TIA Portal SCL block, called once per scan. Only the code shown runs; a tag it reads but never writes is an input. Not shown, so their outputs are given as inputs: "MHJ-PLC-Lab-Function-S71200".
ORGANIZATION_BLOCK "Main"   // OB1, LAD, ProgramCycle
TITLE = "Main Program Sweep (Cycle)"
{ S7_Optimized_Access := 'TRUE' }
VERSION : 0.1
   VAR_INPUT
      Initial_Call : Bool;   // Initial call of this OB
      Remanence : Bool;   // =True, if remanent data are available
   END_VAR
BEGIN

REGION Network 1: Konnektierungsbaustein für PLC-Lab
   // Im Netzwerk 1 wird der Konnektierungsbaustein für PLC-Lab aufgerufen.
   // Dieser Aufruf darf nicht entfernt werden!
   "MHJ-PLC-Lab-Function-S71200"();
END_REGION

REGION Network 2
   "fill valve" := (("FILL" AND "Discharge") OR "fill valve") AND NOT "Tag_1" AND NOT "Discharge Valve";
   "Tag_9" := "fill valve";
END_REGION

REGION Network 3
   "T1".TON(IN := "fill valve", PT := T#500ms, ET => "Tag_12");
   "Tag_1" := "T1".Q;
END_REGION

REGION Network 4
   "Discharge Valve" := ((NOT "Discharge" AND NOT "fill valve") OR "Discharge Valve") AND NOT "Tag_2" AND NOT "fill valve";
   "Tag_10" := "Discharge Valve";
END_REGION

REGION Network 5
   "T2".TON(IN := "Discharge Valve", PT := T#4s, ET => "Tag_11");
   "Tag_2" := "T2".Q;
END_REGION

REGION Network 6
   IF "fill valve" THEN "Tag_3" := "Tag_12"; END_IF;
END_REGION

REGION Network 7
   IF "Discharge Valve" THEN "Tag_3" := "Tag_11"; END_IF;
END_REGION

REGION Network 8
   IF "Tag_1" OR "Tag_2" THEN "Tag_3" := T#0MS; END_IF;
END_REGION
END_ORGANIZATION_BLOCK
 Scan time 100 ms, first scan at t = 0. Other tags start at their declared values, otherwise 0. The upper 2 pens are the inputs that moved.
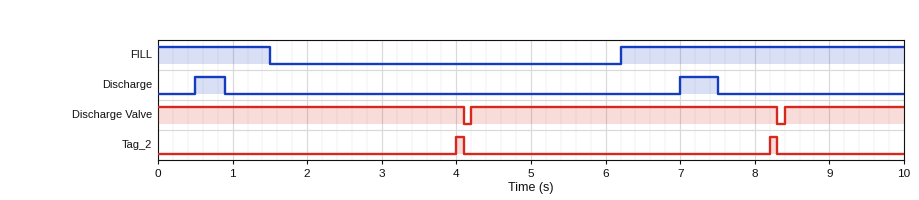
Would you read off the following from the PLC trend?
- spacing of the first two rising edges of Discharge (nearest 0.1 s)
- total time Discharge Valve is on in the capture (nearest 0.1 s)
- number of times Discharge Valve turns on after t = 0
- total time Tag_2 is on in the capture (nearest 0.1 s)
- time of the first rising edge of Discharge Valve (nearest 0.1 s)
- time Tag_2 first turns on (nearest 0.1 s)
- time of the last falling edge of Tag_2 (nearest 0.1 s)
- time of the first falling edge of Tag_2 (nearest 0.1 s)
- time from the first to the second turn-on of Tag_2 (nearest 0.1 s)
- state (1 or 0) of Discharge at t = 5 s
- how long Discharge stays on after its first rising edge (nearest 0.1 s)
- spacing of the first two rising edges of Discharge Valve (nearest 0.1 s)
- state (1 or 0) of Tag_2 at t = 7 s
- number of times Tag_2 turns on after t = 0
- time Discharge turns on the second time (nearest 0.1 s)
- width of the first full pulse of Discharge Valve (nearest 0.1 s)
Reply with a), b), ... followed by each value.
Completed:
a) 6.5 s
b) 9.8 s
c) 2
d) 0.2 s
e) 4.2 s
f) 4.0 s
g) 8.3 s
h) 4.1 s
i) 4.2 s
j) 0
k) 0.4 s
l) 4.2 s
m) 0
n) 2
o) 7.0 s
p) 4.1 s
